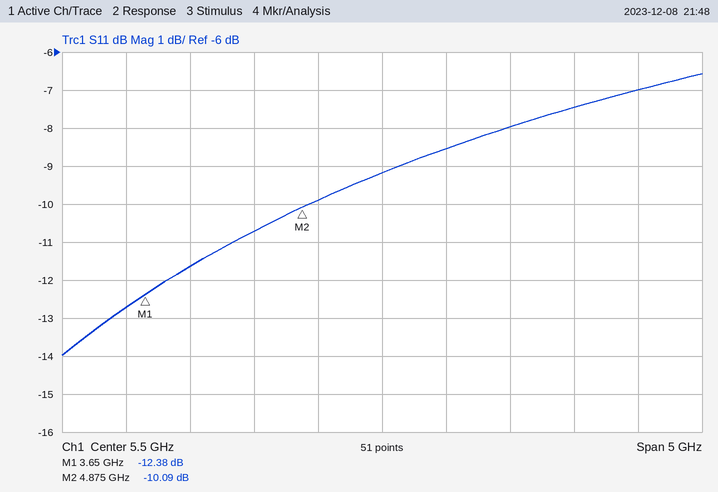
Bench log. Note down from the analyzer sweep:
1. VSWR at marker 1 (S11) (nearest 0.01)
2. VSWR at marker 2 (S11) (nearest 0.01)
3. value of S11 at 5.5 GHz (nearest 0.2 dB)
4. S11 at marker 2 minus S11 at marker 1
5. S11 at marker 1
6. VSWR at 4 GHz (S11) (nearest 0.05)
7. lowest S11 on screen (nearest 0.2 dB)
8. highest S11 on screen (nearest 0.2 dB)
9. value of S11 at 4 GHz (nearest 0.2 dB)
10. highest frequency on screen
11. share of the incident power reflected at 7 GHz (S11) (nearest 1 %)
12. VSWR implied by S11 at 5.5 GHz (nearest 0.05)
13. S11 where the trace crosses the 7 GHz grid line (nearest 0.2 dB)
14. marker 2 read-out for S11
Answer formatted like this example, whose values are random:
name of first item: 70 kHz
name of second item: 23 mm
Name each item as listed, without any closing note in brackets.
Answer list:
VSWR at marker 1 (S11): 1.63
VSWR at marker 2 (S11): 1.91
value of S11 at 5.5 GHz: -9.2 dB
S11 at marker 2 minus S11 at marker 1: 2.29 dB
S11 at marker 1: -12.38 dB
VSWR at 4 GHz (S11): 1.70
lowest S11 on screen: -14.0 dB
highest S11 on screen: -6.6 dB
value of S11 at 4 GHz: -11.6 dB
highest frequency on screen: 8 GHz
share of the incident power reflected at 7 GHz (S11): 18 %
VSWR implied by S11 at 5.5 GHz: 2.05
S11 where the trace crosses the 7 GHz grid line: -7.4 dB
marker 2 read-out for S11: -10.09 dB
